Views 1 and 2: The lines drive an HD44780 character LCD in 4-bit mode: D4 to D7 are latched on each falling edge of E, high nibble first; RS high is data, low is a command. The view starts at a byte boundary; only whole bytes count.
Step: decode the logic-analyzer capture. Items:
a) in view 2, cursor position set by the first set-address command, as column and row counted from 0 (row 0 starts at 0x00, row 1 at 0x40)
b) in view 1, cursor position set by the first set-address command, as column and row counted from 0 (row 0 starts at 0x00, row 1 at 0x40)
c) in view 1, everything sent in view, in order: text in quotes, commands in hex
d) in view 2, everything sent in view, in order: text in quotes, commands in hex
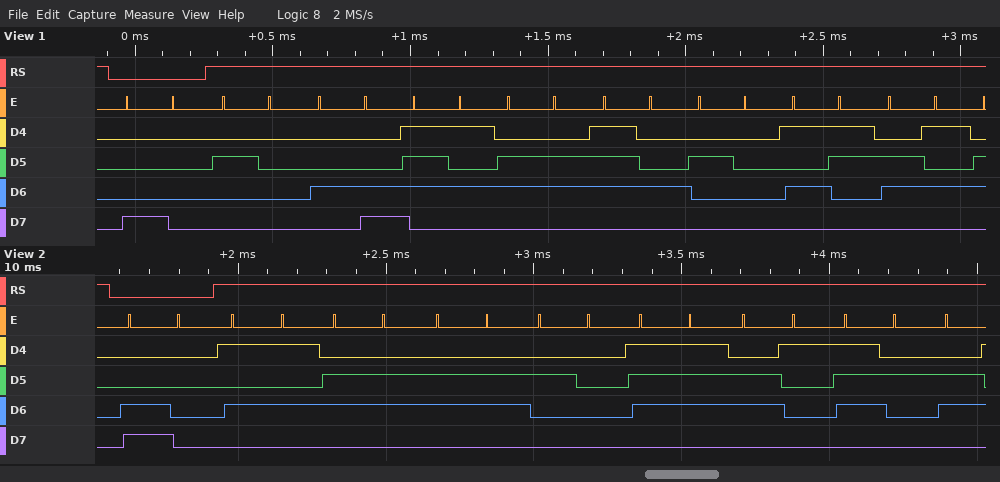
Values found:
column 0, row 1
column 0, row 0
0x80 " Luft Se"
0xC0 "Uff war"
